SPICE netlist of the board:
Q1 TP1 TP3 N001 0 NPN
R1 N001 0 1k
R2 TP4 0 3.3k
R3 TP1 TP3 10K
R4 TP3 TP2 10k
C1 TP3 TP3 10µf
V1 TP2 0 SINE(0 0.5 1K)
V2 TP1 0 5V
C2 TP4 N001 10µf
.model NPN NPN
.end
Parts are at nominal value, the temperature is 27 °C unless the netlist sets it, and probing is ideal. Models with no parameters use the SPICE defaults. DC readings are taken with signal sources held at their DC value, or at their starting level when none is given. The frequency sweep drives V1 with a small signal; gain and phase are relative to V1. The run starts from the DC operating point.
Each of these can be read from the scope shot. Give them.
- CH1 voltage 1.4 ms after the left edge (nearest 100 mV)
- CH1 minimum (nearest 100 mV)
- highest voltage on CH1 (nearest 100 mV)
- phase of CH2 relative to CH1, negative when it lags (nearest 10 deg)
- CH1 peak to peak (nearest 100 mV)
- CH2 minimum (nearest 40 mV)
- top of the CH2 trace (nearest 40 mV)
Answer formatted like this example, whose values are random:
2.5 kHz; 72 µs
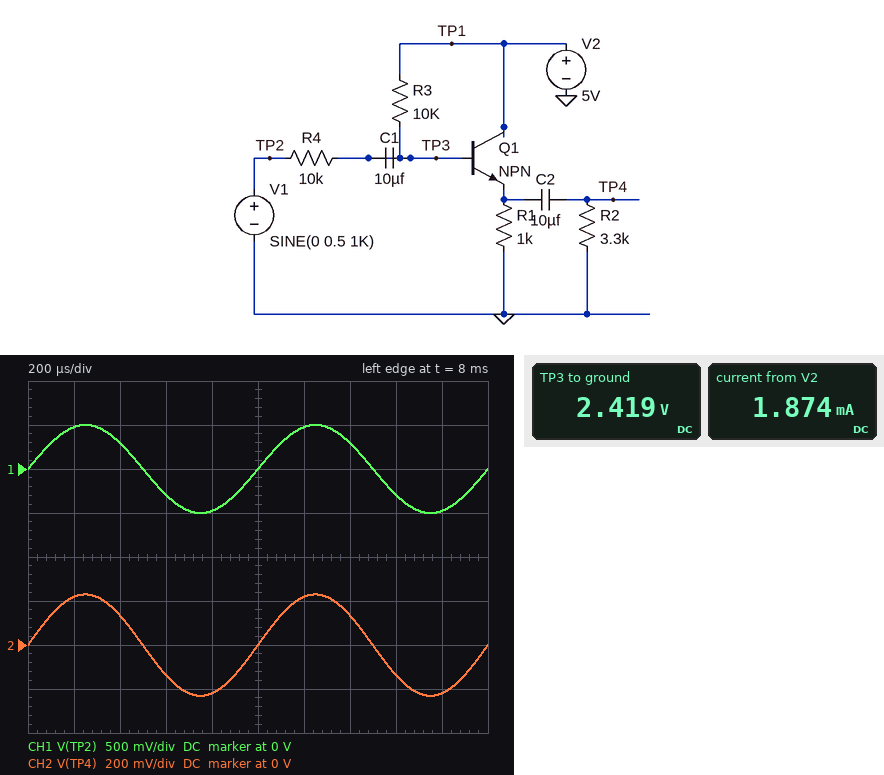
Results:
300 mV; -500 mV; 500 mV; 0 deg; 1.0 V; -240 mV; 240 mV
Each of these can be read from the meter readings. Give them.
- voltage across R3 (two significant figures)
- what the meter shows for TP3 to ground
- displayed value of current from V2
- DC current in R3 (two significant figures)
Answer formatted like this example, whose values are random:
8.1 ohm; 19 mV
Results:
2.6 V; 2.419 V; 1.874 mA; 260 µA
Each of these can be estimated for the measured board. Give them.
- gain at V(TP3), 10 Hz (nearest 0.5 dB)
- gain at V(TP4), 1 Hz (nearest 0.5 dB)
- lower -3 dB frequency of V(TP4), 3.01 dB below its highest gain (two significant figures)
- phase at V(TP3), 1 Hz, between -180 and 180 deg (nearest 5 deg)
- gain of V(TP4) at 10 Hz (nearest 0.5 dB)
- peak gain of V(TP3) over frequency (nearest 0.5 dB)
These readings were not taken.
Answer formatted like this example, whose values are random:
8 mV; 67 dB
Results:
-6.5 dB; -20.5 dB; 4.7 Hz; 0 deg; -7.5 dB; -6.5 dB
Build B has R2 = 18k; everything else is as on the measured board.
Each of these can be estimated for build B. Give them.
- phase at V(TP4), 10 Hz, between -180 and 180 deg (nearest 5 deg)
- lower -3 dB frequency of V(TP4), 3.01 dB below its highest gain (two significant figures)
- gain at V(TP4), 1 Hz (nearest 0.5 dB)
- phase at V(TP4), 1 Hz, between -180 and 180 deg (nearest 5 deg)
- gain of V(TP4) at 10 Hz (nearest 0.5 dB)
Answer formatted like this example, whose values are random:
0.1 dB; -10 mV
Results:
5 deg; 880 mHz; -9.0 dB; 40 deg; -6.5 dB
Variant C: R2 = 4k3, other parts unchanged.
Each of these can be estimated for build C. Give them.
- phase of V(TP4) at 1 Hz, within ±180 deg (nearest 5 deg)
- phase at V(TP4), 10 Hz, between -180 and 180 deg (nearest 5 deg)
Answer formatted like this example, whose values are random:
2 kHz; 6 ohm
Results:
75 deg; 20 deg
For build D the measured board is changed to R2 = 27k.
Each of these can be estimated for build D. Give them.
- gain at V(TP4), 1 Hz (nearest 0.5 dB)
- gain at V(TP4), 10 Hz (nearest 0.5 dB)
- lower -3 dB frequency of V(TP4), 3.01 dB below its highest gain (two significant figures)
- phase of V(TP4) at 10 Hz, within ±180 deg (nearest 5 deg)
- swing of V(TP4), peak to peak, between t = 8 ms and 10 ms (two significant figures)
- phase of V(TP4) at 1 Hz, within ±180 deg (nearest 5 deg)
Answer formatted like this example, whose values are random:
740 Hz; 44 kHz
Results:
-8.0 dB; -6.5 dB; 590 mHz; 5 deg; 470 mV; 30 deg
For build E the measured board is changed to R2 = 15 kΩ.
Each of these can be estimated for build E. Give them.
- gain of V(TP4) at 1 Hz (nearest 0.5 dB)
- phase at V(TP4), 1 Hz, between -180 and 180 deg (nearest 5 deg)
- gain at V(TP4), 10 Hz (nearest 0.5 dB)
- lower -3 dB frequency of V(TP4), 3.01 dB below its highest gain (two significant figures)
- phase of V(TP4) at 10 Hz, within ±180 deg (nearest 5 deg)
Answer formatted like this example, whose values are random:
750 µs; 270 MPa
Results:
-10.0 dB; 45 deg; -6.5 dB; 1.1 Hz; 5 deg
